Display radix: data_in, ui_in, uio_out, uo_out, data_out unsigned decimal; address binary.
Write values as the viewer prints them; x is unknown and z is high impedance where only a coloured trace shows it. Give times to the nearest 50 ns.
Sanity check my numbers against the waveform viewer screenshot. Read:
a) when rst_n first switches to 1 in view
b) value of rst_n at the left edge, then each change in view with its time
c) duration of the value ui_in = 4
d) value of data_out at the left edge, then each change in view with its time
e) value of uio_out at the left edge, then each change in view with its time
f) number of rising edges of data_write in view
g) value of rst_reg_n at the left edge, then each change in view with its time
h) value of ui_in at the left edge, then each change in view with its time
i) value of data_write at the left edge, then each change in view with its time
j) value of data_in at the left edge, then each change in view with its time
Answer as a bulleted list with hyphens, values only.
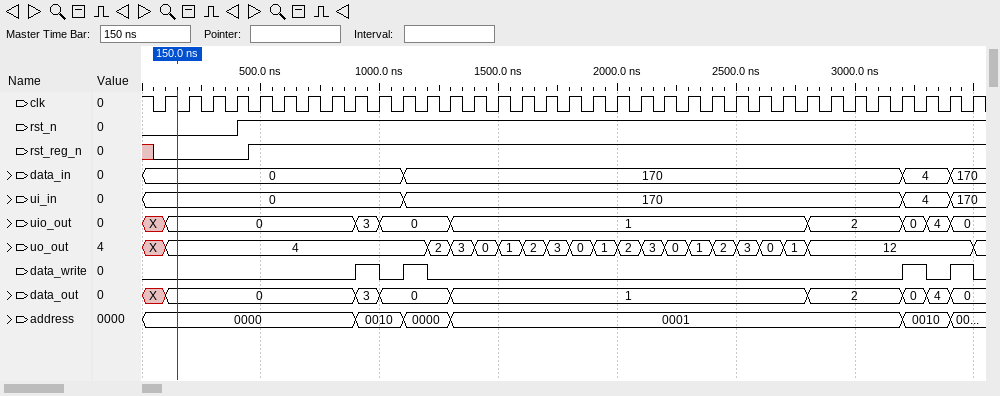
- 400 ns
- 0, 1 at 400 ns
- 200 ns
- X, 0 at 100 ns, 3 at 900 ns, 0 at 1000 ns, 1 at 1300 ns, 2 at 2800 ns, 0 at 3200 ns, 4 at 3300 ns, 0 at 3400 ns
- X, 0 at 100 ns, 3 at 900 ns, 0 at 1000 ns, 1 at 1300 ns, 2 at 2800 ns, 0 at 3200 ns, 4 at 3300 ns, 0 at 3400 ns
- 4
- x, 0 at 50 ns, 1 at 450 ns
- 0, 170 at 1100 ns, 4 at 3200 ns, 170 at 3400 ns
- 0, 1 at 900 ns, 0 at 1000 ns, 1 at 1100 ns, 0 at 1200 ns, 1 at 3200 ns, 0 at 3300 ns, 1 at 3400 ns, 0 at 3500 ns
- 0, 170 at 1100 ns, 4 at 3200 ns, 170 at 3400 ns
